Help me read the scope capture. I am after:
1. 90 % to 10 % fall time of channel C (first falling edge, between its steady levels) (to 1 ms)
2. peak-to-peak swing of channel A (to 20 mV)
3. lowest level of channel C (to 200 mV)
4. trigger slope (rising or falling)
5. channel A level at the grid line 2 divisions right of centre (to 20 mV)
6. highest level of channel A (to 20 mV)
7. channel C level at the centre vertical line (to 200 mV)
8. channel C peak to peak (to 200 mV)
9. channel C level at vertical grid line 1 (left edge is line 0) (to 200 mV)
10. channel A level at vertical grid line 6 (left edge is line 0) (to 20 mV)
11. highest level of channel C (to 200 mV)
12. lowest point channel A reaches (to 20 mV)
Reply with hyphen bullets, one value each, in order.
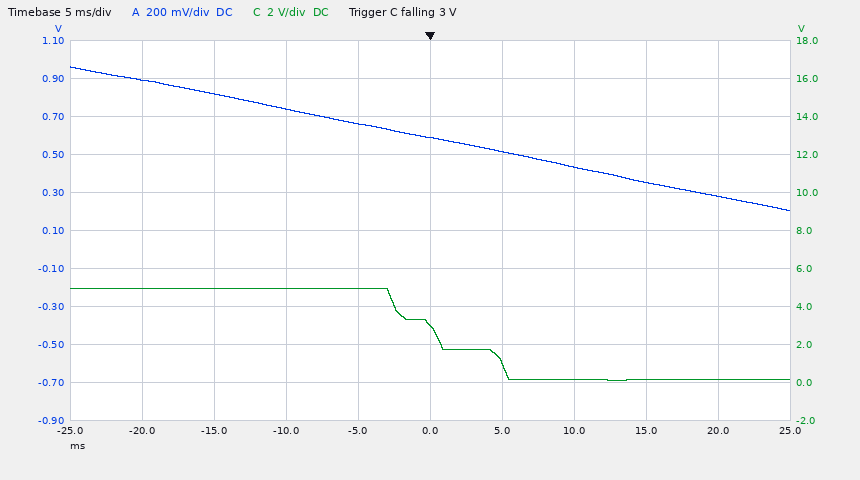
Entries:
- 8 ms
- 760 mV
- 200 mV
- falling
- 440 mV
- 960 mV
- 3.0 V
- 4.8 V
- 5.0 V
- 520 mV
- 5.0 V
- 200 mV
